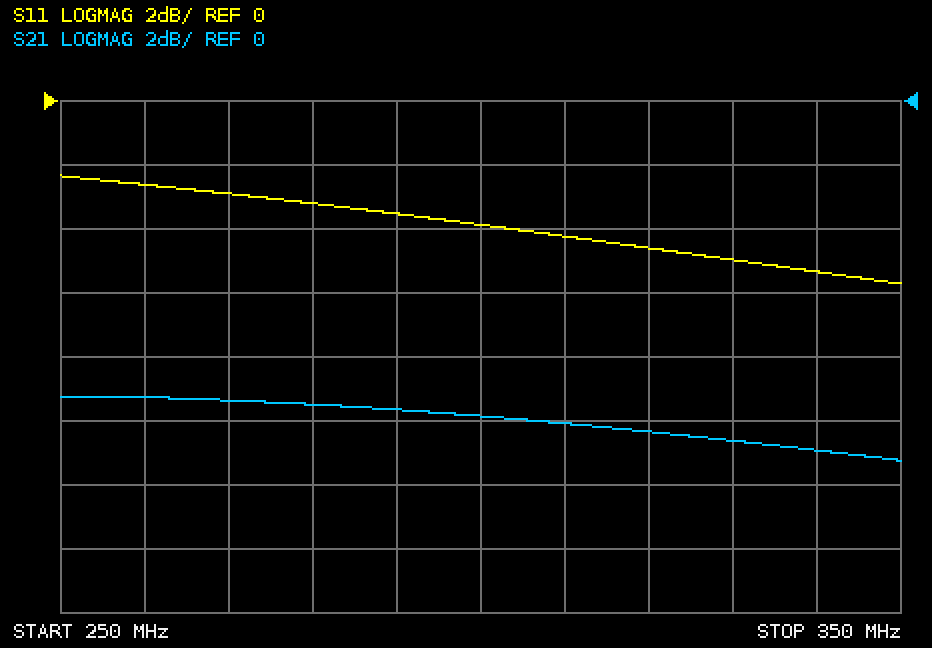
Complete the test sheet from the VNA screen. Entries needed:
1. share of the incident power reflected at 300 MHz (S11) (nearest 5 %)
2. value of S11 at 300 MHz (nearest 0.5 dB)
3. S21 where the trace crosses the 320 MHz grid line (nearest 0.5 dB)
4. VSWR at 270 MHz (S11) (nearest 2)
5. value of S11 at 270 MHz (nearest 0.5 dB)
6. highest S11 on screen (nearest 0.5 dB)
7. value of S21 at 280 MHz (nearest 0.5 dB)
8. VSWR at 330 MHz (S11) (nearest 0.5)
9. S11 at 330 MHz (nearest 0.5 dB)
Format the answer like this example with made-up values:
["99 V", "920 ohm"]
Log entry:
["40 %", "-4.0 dB", "-10.5 dB", "6", "-3.0 dB", "-2.5 dB", "-9.5 dB", "3.5", "-5.0 dB"]
